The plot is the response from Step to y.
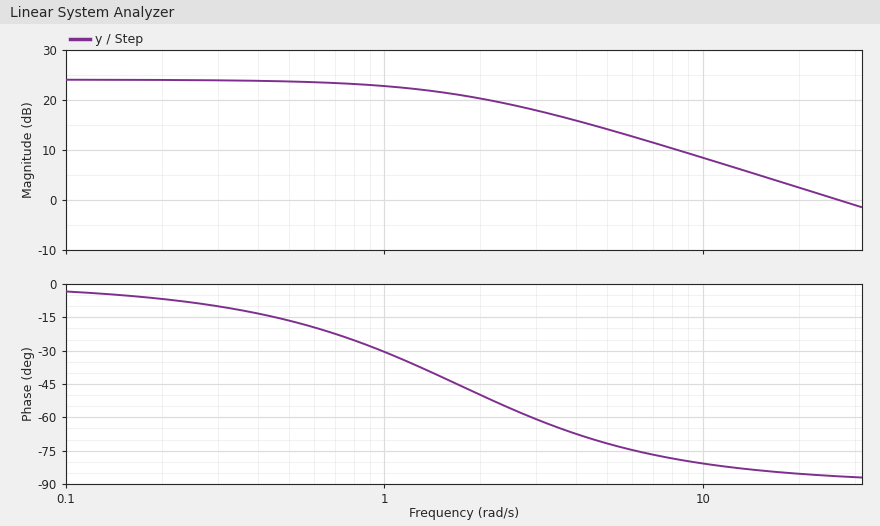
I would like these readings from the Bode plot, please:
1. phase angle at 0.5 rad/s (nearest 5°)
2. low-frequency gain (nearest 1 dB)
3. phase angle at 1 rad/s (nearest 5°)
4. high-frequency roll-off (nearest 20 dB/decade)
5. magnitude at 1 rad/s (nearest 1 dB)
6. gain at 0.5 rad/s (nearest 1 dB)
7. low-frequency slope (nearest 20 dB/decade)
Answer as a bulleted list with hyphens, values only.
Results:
- -15°
- 24 dB
- -30°
- -20 dB/decade
- 23 dB
- 24 dB
- 0 dB/decade
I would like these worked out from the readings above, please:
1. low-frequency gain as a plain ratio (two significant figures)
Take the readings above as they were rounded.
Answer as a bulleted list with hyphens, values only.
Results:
- 16
